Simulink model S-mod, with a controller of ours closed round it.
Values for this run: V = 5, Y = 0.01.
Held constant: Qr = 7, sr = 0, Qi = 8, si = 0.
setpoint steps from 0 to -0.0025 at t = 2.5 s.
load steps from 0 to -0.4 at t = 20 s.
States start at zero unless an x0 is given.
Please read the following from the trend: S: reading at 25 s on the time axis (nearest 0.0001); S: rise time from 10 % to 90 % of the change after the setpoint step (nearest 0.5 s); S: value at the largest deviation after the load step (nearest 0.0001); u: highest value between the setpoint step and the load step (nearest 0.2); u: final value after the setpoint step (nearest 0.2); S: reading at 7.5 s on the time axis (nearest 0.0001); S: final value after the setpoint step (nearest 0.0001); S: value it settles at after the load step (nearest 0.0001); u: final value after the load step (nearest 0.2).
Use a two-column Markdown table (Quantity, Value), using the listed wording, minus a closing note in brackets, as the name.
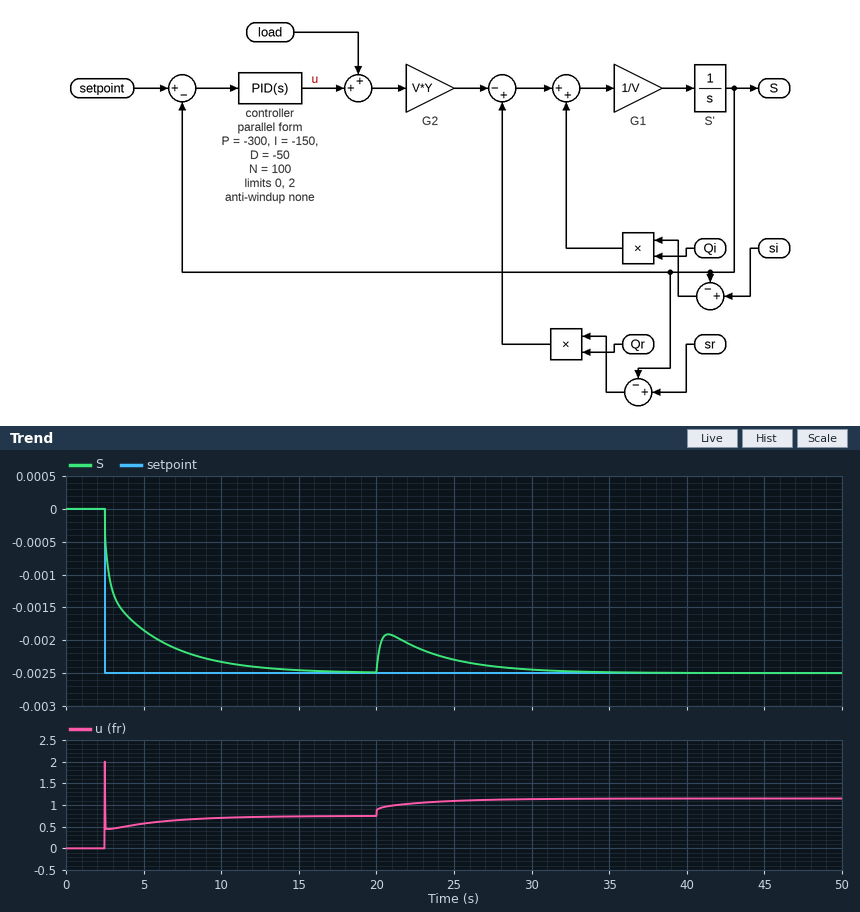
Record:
| Quantity | Value |
|---|---|
| S: reading at 25 s on the time axis | -0.0023 |
| S: rise time from 10 % to 90 % of the change after the setpoint step | 6.0 s |
| S: value at the largest deviation after the load step | -0.0019 |
| u: highest value between the setpoint step and the load step | 2.0 |
| u: final value after the setpoint step | 0.8 |
| S: reading at 7.5 s on the time axis | -0.0022 |
| S: final value after the setpoint step | -0.0025 |
| S: value it settles at after the load step | -0.0025 |
| u: final value after the load step | 1.2 |
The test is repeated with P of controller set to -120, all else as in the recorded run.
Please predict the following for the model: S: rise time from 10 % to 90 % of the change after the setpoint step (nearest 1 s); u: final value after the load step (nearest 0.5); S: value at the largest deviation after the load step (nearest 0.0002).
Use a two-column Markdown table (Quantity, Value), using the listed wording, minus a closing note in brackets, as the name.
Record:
| Quantity | Value |
|---|---|
| S: rise time from 10 % to 90 % of the change after the setpoint step | 5 s |
| u: final value after the load step | 1.0 |
| S: value at the largest deviation after the load step | -0.0018 |
